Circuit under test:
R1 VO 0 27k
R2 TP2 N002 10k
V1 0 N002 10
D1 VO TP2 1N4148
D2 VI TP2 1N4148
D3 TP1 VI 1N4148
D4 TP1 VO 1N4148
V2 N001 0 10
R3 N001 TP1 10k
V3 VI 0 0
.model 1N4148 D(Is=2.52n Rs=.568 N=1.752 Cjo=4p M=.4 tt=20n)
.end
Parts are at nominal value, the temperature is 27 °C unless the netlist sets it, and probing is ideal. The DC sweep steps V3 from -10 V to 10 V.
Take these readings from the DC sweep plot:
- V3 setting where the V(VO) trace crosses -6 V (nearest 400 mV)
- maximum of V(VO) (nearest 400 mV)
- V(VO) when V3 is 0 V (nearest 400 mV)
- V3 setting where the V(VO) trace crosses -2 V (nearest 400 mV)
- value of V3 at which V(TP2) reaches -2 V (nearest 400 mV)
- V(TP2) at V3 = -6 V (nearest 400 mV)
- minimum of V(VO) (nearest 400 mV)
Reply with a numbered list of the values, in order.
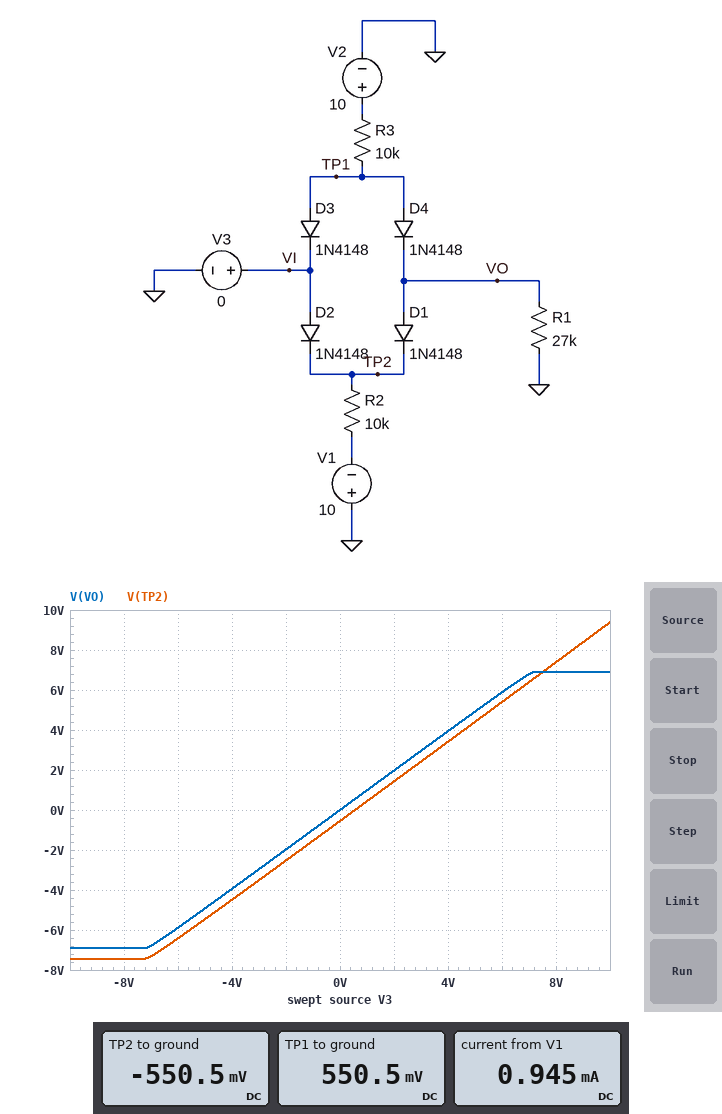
1. -6.0 V
2. 6.8 V
3. 0 V
4. -2.0 V
5. -1.6 V
6. -6.4 V
7. -6.8 V
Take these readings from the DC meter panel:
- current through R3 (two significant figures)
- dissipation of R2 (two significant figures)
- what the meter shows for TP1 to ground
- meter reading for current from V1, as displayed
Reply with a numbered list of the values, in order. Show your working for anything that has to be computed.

1. (10 V - 550.5 mV) / 10 kΩ = 940 µA
2. (-550.5 mV - (-10 V))^2 / 10 kΩ = 8.9 mW
3. 550.5 mV
4. 0.945 mA
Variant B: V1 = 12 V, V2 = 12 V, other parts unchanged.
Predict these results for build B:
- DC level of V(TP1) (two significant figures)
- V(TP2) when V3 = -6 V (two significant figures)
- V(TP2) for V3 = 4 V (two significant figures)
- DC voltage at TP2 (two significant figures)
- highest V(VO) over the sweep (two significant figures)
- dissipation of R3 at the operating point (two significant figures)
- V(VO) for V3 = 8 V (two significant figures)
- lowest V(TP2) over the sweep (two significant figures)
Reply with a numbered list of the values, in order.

1. 560 mV
2. -6.5 V
3. 3.4 V
4. -560 mV
5. 8.4 V
6. 13 mW
7. 7.8 V
8. -8.9 V
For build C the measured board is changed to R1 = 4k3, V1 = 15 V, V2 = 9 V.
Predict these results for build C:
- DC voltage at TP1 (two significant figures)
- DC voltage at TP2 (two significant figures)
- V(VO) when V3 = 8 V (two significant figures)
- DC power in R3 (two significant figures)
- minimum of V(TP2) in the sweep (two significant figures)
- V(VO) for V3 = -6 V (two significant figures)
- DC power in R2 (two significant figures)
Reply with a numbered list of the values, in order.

1. 530 mV
2. -580 mV
3. 2.5 V
4. 7.2 mW
5. -4.9 V
6. -4.3 V
7. 21 mW
